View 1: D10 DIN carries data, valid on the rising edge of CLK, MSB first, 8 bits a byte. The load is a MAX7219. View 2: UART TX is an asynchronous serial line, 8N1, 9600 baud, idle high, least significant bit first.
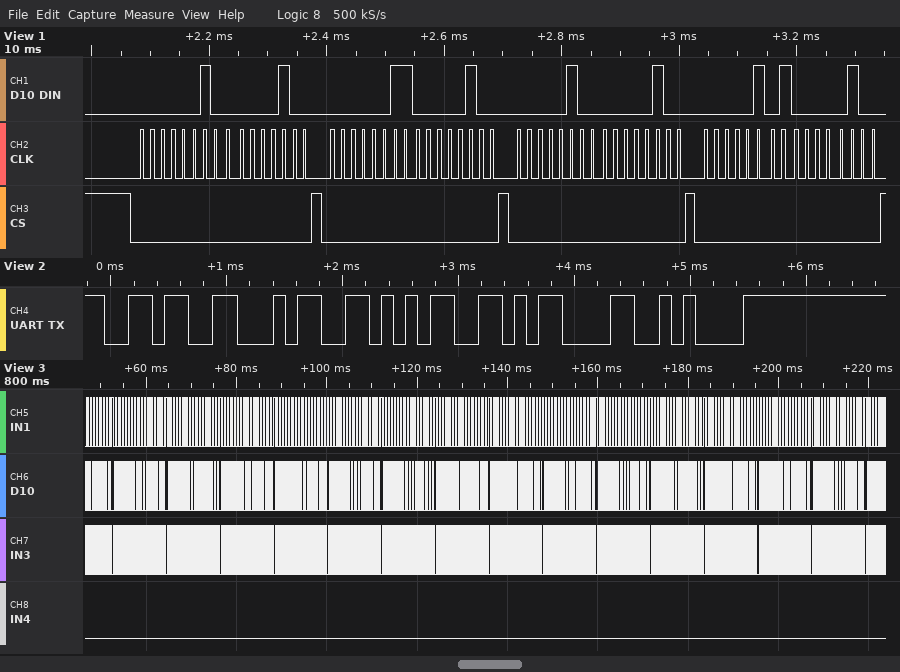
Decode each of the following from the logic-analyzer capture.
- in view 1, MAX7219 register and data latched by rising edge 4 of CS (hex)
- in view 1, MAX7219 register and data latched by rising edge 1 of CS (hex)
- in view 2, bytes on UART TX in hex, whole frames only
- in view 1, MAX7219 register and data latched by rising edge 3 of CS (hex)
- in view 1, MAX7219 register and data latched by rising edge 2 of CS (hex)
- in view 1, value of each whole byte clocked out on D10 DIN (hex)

register 0x5, data 0x04
register 0x2, data 0x04
36 34 35 0D 0A
register 0x4, data 0x04
register 0x3, data 0x04
02 04 03 04 04 04 05 04
